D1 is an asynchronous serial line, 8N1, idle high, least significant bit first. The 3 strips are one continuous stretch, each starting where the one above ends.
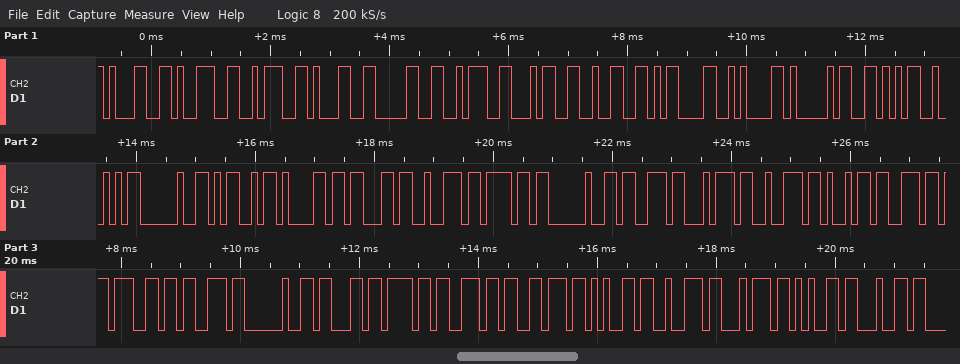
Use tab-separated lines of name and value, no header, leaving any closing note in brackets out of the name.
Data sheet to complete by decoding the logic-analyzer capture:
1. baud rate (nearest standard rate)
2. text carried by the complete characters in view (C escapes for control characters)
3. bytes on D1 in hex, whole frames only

baud rate	9600 baud
text carried by the complete characters in view	"19:10:42\r\nAVR Macro strings converted"
bytes on D1 in hex, whole frames only	31 39 3A 31 30 3A 34 32 0D 0A 41 56 52 20 4D 61 63 72 6F 20 73 74 72 69 6E 67 73 20 63 6F 6E 76 65 72 74 65 64
